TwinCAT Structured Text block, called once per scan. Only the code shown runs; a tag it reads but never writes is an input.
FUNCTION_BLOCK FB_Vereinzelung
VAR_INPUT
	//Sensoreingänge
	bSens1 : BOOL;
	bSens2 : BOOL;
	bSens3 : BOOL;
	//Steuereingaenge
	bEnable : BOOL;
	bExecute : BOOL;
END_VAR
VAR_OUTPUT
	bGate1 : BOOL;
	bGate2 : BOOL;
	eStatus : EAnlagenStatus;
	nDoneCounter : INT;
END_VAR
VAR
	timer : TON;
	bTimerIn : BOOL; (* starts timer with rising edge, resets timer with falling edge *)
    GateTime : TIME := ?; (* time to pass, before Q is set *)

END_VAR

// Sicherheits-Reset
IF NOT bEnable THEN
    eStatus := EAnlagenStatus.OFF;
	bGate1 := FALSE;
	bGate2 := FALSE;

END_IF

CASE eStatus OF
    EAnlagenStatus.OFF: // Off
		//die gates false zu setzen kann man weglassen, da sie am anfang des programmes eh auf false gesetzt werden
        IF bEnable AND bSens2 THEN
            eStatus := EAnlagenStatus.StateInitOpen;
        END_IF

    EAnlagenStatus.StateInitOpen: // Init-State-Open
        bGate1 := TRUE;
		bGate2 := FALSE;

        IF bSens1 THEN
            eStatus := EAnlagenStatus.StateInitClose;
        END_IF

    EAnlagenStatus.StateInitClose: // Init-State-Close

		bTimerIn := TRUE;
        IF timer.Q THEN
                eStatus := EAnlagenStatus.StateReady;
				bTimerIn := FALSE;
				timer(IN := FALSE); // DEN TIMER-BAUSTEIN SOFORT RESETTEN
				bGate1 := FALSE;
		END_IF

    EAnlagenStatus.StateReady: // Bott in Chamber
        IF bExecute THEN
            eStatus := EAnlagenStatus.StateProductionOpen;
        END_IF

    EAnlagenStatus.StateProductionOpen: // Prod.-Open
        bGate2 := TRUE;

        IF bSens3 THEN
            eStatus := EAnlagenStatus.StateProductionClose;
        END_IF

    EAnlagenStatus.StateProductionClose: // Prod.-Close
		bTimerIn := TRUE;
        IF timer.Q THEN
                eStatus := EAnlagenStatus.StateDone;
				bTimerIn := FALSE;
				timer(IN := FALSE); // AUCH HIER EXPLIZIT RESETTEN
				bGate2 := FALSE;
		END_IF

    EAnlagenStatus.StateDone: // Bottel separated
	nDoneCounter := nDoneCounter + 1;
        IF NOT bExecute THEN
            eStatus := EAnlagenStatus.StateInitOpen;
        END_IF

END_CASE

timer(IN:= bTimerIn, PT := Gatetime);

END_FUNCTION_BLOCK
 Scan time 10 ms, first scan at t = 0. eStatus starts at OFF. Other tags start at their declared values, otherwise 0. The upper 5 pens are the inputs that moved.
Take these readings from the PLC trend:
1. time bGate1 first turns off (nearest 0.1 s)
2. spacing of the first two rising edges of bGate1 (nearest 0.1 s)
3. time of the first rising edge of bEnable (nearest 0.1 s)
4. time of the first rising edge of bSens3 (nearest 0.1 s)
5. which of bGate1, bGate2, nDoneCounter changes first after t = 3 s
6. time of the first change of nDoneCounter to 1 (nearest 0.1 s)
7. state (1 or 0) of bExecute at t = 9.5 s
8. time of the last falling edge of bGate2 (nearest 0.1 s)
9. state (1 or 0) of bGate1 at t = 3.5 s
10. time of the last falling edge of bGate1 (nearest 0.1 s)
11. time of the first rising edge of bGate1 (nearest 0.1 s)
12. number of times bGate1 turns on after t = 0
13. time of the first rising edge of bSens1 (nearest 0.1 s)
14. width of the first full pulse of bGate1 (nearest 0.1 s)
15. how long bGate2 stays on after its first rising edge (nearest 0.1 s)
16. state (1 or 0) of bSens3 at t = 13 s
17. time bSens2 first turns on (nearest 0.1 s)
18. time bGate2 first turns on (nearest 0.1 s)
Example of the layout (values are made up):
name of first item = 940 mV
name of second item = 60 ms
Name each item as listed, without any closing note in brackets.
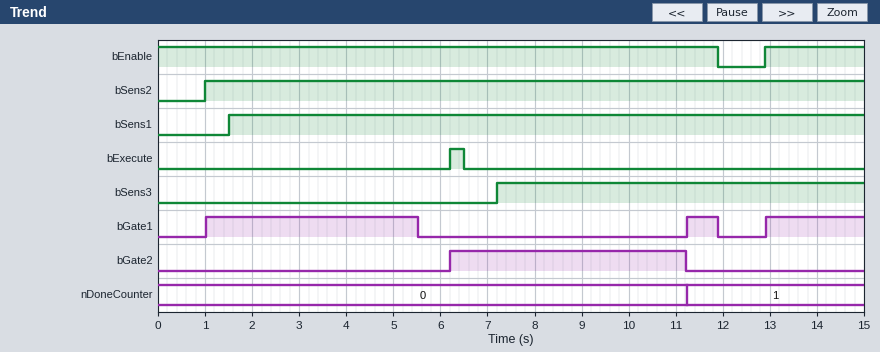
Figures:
time bGate1 first turns off = 5.5 s
spacing of the first two rising edges of bGate1 = 10.2 s
time of the first rising edge of bEnable = 12.9 s
time of the first rising edge of bSens3 = 7.2 s
which of bGate1, bGate2, nDoneCounter changes first after t = 3 s = bGate1
time of the first change of nDoneCounter to 1 = 11.2 s
state (1 or 0) of bExecute at t = 9.5 s = 0
time of the last falling edge of bGate2 = 11.2 s
state (1 or 0) of bGate1 at t = 3.5 s = 1
time of the last falling edge of bGate1 = 11.9 s
time of the first rising edge of bGate1 = 1.0 s
number of times bGate1 turns on after t = 0 = 3
time of the first rising edge of bSens1 = 1.5 s
width of the first full pulse of bGate1 = 4.5 s
how long bGate2 stays on after its first rising edge = 5.0 s
state (1 or 0) of bSens3 at t = 13 s = 1
time bSens2 first turns on = 1.0 s
time bGate2 first turns on = 6.2 s
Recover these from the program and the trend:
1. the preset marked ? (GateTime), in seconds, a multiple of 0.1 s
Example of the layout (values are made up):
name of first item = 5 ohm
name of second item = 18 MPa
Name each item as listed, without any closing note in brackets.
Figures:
the preset marked ? (GateTime), in seconds, a multiple of 0.1 s = 4.0 s
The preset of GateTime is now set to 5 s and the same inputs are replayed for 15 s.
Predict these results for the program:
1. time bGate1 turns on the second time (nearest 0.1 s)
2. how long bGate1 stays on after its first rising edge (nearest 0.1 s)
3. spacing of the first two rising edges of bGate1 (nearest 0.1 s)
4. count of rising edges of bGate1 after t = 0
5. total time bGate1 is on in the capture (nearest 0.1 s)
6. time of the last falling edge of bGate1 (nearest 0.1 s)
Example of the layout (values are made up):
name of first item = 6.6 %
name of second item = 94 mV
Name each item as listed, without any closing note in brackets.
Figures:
time bGate1 turns on the second time = 12.9 s
how long bGate1 stays on after its first rising edge = 5.5 s
spacing of the first two rising edges of bGate1 = 11.9 s
count of rising edges of bGate1 after t = 0 = 2
total time bGate1 is on in the capture = 7.6 s
time of the last falling edge of bGate1 = 6.5 s
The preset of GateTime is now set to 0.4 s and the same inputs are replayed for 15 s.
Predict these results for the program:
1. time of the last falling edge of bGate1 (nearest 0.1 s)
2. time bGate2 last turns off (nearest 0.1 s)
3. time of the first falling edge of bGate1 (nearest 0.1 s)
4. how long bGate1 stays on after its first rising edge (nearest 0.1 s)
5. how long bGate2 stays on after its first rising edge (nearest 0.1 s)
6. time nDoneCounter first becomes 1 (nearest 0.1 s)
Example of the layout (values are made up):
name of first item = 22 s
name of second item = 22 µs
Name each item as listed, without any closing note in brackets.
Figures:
time of the last falling edge of bGate1 = 13.3 s
time bGate2 last turns off = 7.6 s
time of the first falling edge of bGate1 = 1.9 s
how long bGate1 stays on after its first rising edge = 0.9 s
how long bGate2 stays on after its first rising edge = 1.4 s
time nDoneCounter first becomes 1 = 7.6 s
